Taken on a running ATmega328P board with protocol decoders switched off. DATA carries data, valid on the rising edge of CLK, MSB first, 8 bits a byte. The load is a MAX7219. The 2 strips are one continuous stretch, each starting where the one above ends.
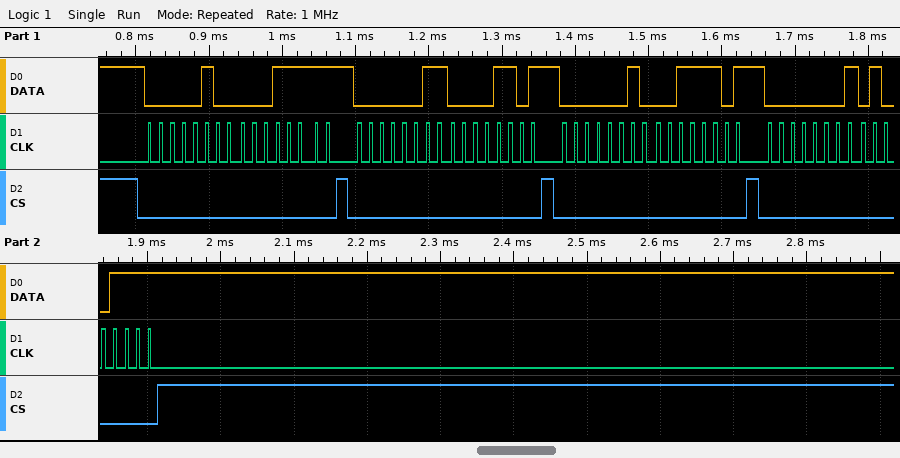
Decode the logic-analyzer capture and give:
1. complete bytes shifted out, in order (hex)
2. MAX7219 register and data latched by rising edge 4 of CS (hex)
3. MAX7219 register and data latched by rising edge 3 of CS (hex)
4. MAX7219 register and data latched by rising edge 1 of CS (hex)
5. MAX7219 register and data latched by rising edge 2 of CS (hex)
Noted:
04 1F 03 0D 02 3D 01 4F
register 0x1, data 0x4F
register 0x2, data 0x3D
register 0x4, data 0x1F
register 0x3, data 0x0D
